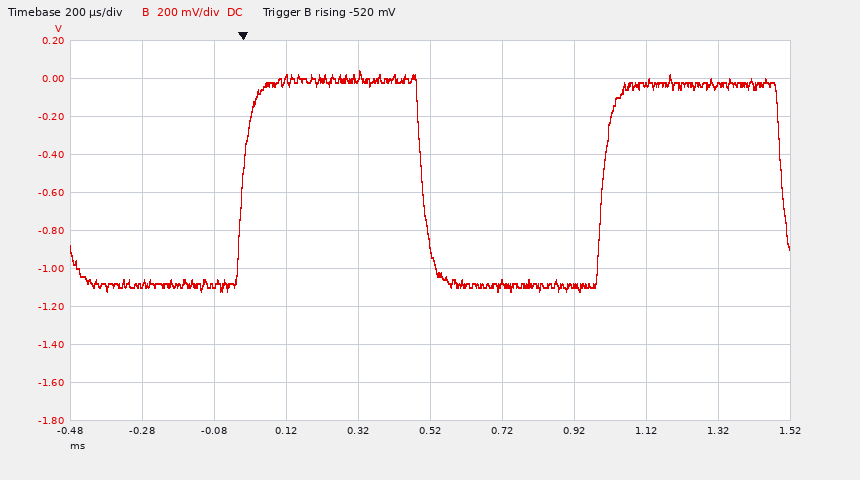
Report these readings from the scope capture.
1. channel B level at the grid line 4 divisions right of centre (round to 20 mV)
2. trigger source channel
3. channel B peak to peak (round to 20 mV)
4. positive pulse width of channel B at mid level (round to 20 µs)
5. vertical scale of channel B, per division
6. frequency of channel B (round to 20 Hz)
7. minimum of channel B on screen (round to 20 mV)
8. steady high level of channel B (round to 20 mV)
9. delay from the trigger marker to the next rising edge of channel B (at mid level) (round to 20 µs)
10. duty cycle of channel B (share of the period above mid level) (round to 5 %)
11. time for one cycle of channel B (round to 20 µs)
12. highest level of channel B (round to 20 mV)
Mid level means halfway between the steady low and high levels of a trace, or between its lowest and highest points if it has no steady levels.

-40 mV
channel B
1.16 V
500 µs
200 mV
1.00 kHz
-1.12 V
-20 mV
1.00 ms
50 %
1.00 ms
40 mV
